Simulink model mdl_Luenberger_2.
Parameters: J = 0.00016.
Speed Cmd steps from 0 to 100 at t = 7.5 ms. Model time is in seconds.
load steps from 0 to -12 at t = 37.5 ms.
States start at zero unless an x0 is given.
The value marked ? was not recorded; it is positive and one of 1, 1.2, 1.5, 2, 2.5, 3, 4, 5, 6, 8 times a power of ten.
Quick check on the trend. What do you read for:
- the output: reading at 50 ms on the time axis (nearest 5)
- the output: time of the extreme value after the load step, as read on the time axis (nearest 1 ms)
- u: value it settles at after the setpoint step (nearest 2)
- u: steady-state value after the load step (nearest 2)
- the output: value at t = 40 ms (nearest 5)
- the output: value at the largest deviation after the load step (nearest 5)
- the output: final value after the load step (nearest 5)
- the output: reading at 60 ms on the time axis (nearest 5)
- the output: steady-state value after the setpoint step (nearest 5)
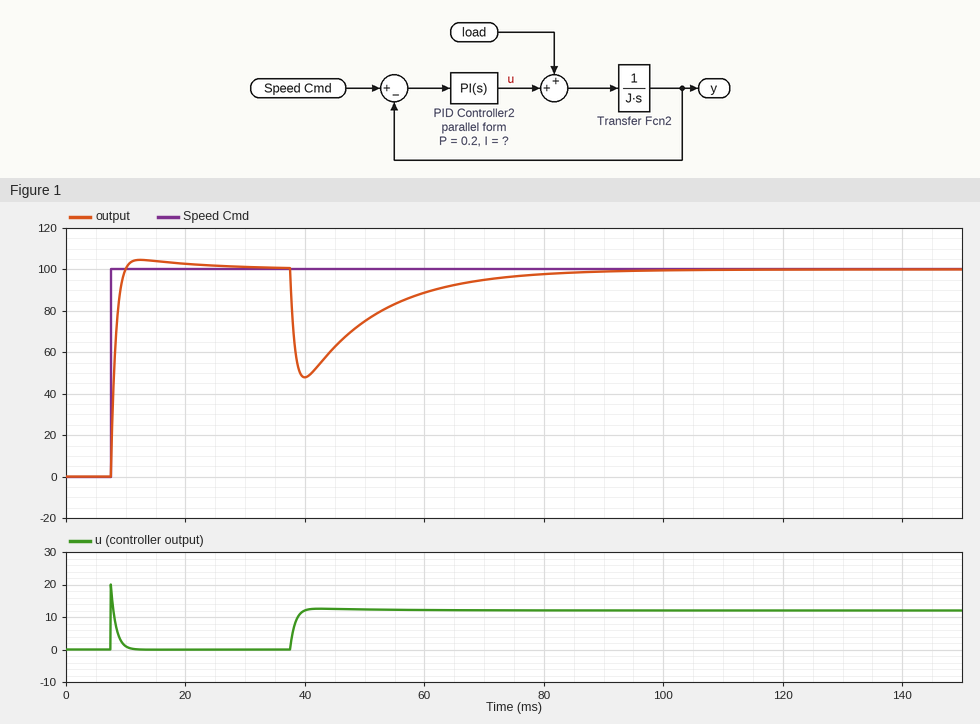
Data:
75
40 ms
0
12
50
50
100
90
100
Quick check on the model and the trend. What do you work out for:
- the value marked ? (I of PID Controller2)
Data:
15
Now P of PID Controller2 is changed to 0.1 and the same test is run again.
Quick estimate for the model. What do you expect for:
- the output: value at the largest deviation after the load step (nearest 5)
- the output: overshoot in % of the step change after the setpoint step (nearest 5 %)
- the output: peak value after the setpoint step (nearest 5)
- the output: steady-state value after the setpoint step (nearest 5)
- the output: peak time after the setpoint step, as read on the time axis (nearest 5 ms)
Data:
10
15 %
115
100
15 ms
